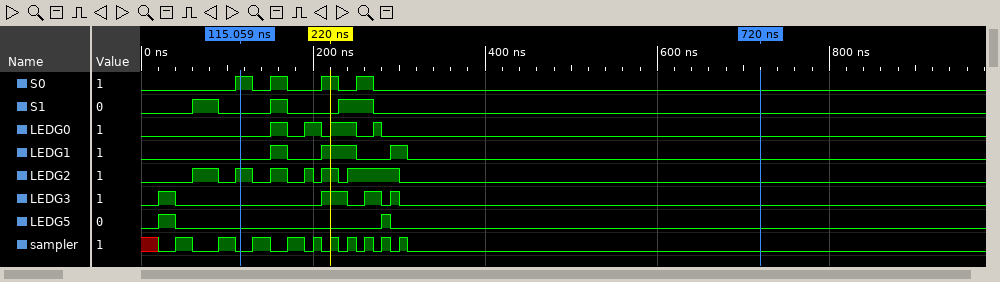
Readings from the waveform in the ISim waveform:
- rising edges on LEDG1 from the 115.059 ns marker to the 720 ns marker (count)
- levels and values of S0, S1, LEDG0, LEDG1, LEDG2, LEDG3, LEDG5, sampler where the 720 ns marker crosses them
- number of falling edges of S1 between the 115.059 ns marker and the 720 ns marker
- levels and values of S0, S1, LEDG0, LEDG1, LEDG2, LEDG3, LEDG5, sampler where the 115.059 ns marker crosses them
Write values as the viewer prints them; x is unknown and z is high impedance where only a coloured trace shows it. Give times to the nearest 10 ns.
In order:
3
S0=0, S1=0, LEDG0=0, LEDG1=0, LEDG2=0, LEDG3=0, LEDG5=0, sampler=0
2
S0=1, S1=0, LEDG0=0, LEDG1=0, LEDG2=1, LEDG3=0, LEDG5=0, sampler=0
